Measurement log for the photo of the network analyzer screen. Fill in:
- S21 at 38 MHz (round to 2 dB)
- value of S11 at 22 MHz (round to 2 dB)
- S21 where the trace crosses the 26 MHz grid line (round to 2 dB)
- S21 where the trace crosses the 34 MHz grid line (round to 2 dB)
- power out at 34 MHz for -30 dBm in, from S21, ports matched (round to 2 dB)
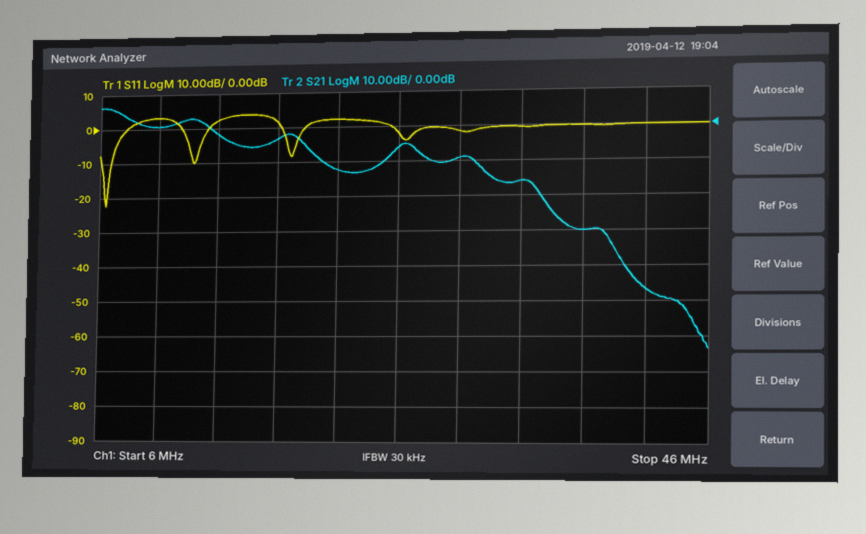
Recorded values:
-30 dB
2 dB
-6 dB
-16 dB
-46 dBm
